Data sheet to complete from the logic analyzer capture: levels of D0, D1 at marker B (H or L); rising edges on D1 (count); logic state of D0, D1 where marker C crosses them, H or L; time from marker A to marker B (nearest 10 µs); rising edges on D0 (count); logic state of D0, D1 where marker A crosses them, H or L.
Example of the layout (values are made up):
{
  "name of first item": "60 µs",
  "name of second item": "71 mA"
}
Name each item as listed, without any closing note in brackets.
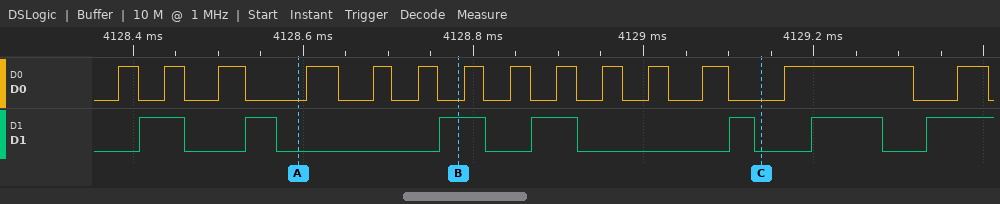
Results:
{
  "levels of D0, D1 at marker B": "D0=L, D1=H",
  "rising edges on D1": "7",
  "logic state of D0, D1 where marker C crosses them, H or L": "D0=L, D1=L",
  "time from marker A to marker B": "190 µs",
  "rising edges on D0": "14",
  "logic state of D0, D1 where marker A crosses them, H or L": "D0=L, D1=L"
}
